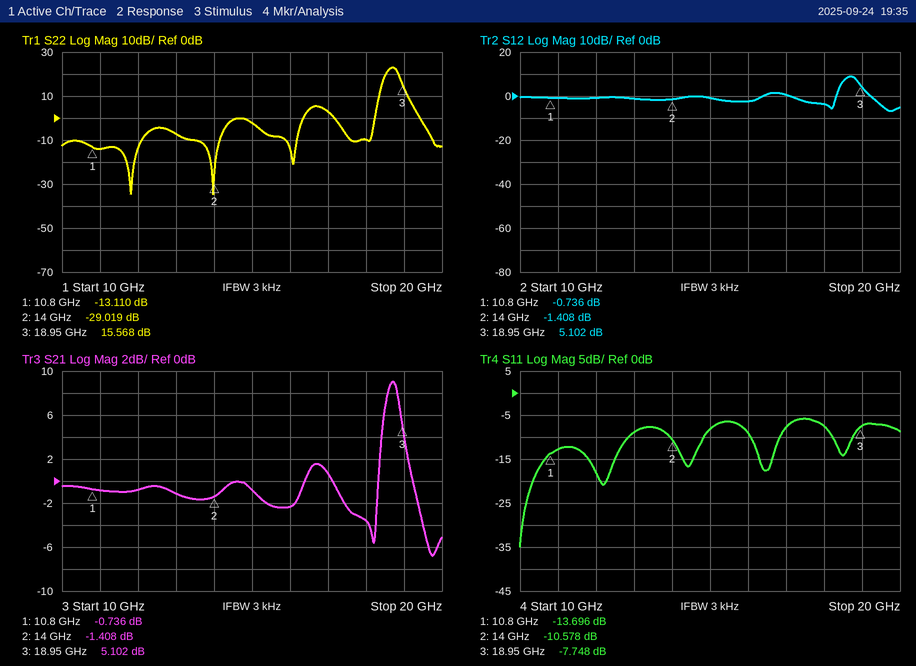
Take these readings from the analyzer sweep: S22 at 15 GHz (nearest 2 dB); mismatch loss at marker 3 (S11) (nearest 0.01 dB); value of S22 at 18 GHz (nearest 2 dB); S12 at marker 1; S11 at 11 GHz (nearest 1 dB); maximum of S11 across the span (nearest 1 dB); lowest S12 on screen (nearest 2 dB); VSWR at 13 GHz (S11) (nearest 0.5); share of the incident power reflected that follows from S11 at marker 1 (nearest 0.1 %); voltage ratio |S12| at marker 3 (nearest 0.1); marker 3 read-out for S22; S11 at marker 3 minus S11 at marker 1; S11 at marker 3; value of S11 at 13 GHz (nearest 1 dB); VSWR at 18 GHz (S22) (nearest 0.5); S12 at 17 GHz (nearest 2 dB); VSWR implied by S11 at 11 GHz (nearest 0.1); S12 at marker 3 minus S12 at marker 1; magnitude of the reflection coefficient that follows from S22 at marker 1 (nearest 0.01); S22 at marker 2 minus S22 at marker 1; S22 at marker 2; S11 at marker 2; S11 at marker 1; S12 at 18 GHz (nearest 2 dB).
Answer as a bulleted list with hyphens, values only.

- -2 dB
- 0.80 dB
- -10 dB
- -0.736 dB
- -13 dB
- -6 dB
- -6 dB
- 2.0
- 4.3 %
- 1.8
- 15.568 dB
- 5.948 dB
- -7.748 dB
- -9 dB
- 2.0
- 0 dB
- 1.6
- 5.838 dB
- 0.22
- -15.909 dB
- -29.019 dB
- -10.578 dB
- -13.696 dB
- -4 dB
